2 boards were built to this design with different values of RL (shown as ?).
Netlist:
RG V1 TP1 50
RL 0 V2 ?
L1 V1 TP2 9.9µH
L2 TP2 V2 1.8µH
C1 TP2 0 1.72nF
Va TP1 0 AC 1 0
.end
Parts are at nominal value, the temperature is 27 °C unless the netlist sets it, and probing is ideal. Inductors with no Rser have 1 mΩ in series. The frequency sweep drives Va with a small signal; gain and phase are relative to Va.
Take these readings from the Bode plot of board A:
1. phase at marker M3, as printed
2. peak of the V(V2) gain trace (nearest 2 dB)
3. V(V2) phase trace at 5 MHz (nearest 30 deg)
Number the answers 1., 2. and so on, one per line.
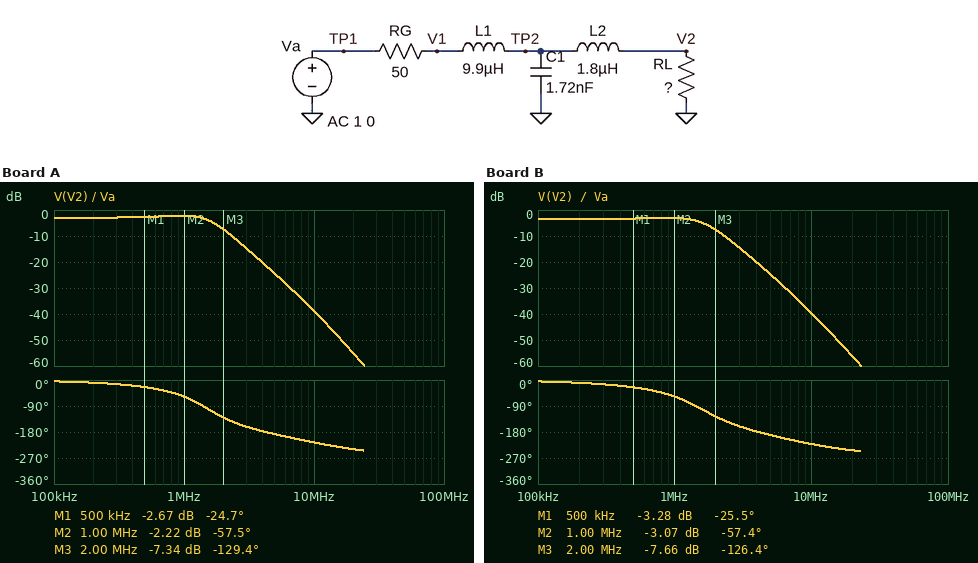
1. -129.4 deg
2. -2 dB
3. -180 deg
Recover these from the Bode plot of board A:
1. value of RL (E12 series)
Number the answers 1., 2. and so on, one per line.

1. 120 Ω
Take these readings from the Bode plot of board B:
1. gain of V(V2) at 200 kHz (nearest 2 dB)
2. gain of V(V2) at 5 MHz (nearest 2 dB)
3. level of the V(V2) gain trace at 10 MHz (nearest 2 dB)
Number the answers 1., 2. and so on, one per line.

1. -4 dB
2. -24 dB
3. -40 dB
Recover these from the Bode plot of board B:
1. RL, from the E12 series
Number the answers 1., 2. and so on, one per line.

1. 100 Ω
